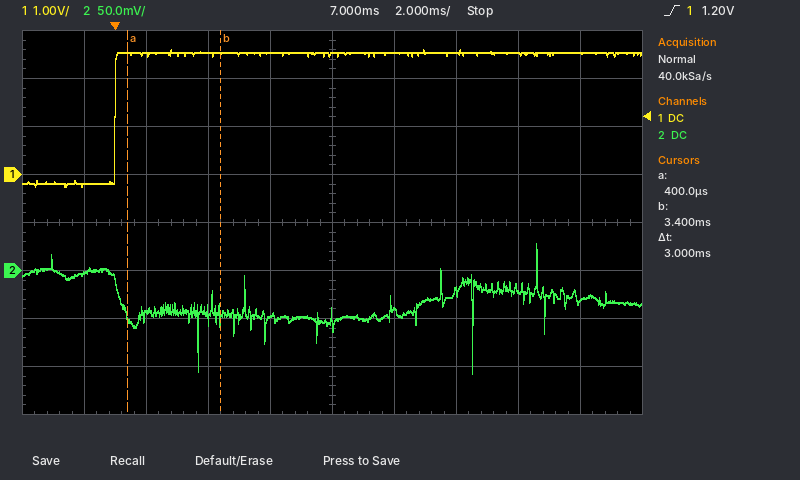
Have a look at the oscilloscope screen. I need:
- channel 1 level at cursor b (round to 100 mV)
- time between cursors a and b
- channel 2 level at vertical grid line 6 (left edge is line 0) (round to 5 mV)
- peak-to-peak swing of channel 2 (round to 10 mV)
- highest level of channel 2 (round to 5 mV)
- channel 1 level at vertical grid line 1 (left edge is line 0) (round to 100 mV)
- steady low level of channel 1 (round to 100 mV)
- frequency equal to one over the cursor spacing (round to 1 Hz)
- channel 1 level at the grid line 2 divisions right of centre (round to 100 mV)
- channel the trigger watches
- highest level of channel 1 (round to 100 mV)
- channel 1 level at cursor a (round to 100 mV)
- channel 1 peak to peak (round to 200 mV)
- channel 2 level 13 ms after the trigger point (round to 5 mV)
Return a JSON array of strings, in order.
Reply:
["2.5 V", "3 ms", "-40 mV", "140 mV", "30 mV", "-200 mV", "-200 mV", "333 Hz", "2.5 V", "channel 1", "2.6 V", "2.5 V", "2.8 V", "-20 mV"]
